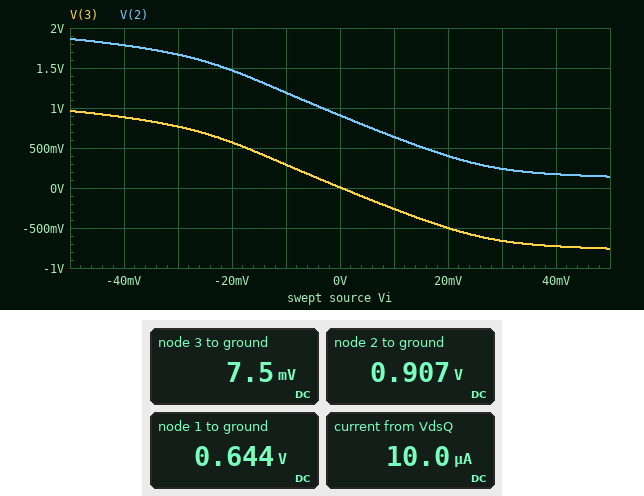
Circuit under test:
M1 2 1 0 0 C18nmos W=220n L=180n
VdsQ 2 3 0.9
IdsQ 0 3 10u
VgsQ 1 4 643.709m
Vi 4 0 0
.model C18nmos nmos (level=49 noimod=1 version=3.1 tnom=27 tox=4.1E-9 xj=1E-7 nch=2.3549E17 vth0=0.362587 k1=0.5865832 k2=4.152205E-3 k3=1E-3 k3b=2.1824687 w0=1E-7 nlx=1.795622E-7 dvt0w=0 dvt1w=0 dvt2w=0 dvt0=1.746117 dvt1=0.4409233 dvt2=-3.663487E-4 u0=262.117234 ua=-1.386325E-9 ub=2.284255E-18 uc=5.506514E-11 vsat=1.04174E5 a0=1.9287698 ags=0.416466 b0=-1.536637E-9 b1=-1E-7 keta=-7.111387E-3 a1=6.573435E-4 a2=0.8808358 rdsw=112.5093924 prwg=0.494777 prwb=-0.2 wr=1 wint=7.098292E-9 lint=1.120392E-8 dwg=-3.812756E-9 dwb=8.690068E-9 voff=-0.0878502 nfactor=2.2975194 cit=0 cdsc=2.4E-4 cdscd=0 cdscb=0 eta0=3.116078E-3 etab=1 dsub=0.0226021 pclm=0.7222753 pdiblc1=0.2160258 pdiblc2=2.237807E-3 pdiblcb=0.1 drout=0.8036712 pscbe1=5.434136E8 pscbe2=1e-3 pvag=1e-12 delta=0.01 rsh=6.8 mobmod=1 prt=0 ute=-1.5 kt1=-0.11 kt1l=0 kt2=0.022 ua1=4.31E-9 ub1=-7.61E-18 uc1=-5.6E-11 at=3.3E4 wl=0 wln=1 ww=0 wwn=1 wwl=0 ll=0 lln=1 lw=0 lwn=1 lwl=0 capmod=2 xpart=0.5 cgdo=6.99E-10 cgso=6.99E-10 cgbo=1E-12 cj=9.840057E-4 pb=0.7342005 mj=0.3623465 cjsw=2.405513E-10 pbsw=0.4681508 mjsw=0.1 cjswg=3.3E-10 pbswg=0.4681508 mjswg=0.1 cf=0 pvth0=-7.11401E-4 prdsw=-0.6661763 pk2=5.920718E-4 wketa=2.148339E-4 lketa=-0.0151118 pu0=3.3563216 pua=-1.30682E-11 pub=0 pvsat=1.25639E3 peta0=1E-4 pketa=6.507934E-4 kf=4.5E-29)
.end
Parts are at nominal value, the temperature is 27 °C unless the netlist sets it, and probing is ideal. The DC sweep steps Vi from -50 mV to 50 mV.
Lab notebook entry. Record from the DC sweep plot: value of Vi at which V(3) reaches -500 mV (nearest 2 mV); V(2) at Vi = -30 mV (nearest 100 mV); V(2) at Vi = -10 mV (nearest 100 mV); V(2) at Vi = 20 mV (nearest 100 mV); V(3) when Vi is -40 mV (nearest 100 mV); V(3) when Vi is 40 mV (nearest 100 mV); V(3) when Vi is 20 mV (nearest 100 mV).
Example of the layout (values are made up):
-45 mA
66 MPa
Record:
20 mV
1.7 V
1.2 V
400 mV
900 mV
-700 mV
-500 mV
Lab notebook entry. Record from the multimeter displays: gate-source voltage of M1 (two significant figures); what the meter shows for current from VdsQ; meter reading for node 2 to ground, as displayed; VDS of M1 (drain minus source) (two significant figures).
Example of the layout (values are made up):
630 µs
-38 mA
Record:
640 mV
10.0 µA
0.907 V
910 mV
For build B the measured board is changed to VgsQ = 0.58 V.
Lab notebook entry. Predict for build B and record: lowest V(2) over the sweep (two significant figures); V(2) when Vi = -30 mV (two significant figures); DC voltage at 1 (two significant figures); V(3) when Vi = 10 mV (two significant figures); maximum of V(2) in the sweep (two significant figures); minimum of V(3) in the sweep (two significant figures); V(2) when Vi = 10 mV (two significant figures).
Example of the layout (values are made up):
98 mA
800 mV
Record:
1.3 V
2.1 V
580 mV
990 mV
2.2 V
400 mV
1.9 V
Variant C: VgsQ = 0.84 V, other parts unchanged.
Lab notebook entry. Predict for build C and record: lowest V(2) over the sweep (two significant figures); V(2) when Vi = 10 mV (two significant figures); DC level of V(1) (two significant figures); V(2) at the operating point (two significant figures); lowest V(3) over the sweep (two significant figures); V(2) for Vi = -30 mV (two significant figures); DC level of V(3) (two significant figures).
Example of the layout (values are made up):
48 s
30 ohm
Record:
50 mV
56 mV
840 mV
58 mV
-850 mV
65 mV
-840 mV
